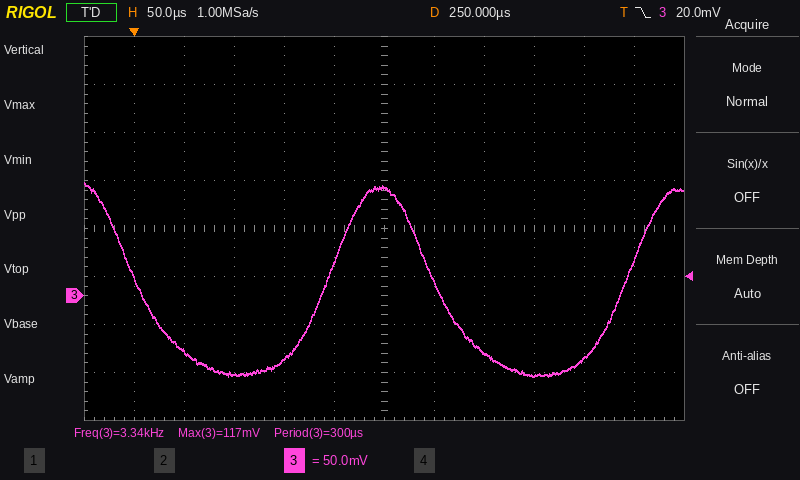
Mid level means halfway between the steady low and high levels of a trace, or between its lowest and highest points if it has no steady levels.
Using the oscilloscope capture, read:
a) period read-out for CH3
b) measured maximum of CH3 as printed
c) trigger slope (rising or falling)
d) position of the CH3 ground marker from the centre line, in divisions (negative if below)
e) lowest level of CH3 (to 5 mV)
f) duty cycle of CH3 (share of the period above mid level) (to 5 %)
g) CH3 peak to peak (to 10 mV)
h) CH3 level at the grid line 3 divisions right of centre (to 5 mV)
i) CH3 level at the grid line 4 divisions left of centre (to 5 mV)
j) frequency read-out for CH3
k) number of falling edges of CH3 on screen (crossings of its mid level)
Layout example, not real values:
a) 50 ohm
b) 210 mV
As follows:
a) 300 µs
b) 117 mV
c) falling
d) -1.4 div
e) -85 mV
f) 35 %
g) 200 mV
h) -85 mV
i) -60 mV
j) 3.34 kHz
k) 2
